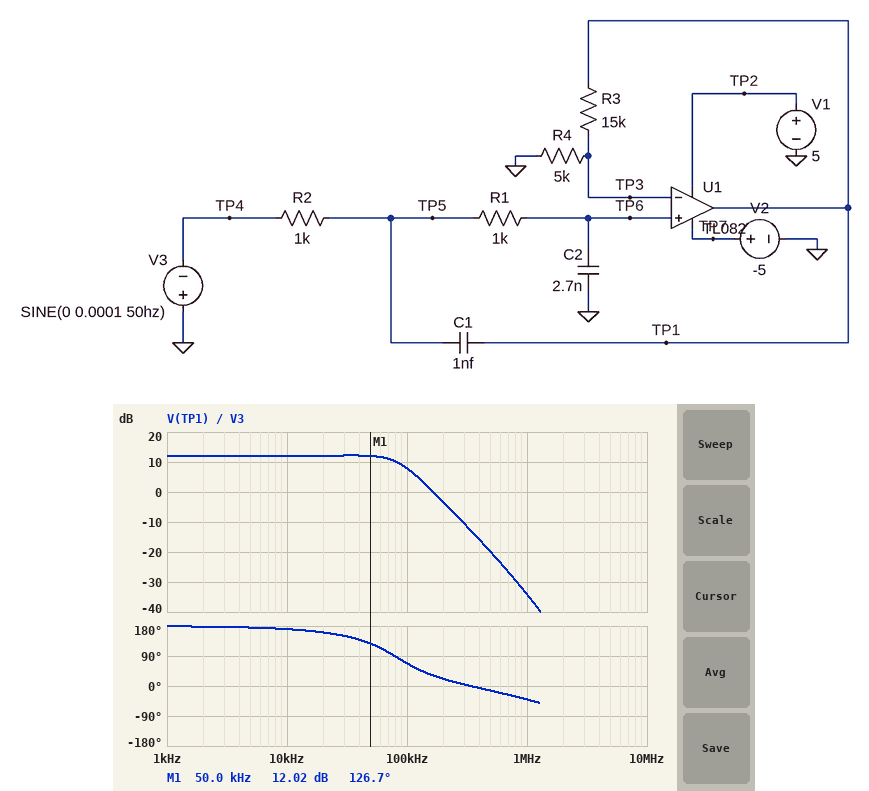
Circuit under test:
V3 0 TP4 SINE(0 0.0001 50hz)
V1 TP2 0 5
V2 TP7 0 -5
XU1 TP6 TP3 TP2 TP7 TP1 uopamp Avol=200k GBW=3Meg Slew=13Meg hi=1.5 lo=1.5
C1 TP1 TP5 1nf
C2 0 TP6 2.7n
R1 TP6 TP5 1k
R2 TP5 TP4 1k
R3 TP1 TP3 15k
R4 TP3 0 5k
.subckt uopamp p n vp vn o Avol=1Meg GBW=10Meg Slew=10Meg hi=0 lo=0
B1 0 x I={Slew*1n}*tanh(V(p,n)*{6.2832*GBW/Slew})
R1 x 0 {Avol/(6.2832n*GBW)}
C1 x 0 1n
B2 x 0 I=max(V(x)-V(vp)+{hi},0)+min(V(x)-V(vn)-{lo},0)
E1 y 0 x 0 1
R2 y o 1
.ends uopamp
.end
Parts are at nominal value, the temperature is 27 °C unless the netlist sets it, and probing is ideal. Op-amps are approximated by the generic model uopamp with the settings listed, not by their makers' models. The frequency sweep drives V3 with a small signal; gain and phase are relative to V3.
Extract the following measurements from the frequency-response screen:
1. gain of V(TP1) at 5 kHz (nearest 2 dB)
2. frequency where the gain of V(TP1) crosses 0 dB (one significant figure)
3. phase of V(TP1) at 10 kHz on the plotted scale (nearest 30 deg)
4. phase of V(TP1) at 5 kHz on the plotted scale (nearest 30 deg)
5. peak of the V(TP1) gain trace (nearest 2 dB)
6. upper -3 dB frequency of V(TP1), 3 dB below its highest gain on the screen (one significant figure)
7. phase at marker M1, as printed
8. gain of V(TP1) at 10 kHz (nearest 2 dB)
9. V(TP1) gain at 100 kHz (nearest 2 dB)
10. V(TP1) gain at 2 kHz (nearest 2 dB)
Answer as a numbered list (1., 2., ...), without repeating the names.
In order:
1. 12 dB
2. 200 kHz
3. 180 deg
4. 180 deg
5. 12 dB
6. 90 kHz
7. 126.7 deg
8. 12 dB
9. 8 dB
10. 12 dB
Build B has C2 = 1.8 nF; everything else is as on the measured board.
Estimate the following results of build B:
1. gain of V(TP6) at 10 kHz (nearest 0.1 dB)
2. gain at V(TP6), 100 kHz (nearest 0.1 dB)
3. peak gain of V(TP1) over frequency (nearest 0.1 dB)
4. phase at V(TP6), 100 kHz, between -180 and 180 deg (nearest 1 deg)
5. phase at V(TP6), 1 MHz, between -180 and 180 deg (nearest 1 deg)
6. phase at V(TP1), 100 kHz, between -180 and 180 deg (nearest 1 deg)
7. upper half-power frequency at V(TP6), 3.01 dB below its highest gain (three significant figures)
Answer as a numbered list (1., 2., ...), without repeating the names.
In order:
1. 0.1 dB
2. 7.5 dB
3. 20.0 dB
4. 85 deg
5. 14 deg
6. 77 deg
7. 112 kHz
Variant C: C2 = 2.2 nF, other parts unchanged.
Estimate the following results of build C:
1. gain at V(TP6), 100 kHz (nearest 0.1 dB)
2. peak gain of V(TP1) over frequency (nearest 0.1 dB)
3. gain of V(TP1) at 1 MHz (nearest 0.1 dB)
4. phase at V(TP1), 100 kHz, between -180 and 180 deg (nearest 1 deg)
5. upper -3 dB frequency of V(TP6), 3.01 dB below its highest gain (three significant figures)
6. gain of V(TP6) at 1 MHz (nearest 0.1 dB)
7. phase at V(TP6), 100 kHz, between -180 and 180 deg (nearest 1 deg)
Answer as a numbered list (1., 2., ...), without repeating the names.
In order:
1. 0.5 dB
2. 14.5 dB
3. -32.5 dB
4. 70 deg
5. 107 kHz
6. -40.1 dB
7. 78 deg
